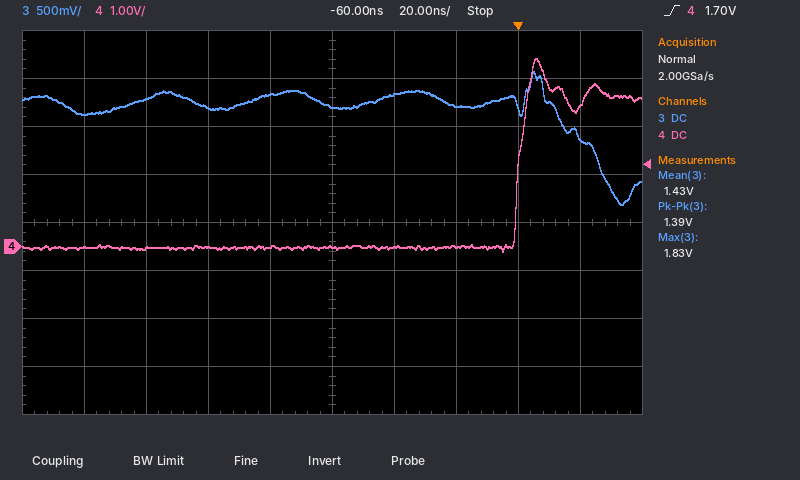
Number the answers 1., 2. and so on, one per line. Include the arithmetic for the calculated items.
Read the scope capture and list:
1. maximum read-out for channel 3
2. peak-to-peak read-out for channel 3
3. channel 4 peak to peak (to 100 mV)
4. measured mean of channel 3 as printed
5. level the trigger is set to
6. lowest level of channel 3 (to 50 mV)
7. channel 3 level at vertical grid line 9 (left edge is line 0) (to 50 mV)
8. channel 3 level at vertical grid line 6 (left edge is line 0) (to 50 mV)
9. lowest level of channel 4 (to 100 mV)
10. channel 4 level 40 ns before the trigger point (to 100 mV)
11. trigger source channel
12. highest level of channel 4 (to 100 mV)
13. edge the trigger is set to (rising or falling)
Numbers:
1. 1.83 V
2. 1.39 V
3. 3.9 V − (-100 mV) = 4.0 V
4. 1.43 V
5. 1.70 V
6. 450 mV
7. 1.15 V
8. 1.60 V
9. -100 mV
10. 0.0 V
11. channel 4
12. 3.9 V
13. rising
